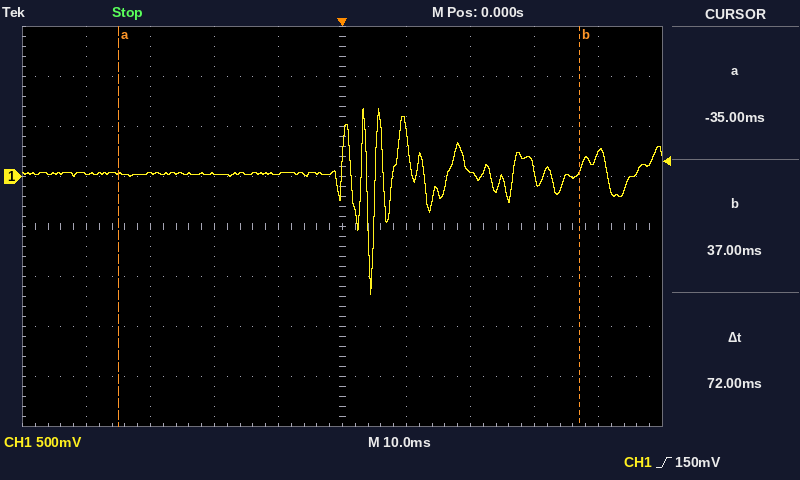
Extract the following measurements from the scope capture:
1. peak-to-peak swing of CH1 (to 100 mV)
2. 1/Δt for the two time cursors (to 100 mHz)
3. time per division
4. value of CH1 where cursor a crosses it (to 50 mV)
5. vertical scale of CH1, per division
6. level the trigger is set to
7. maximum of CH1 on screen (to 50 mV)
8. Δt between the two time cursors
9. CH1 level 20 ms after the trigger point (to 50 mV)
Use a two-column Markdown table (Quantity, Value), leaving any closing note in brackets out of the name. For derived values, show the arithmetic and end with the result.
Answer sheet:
| Quantity | Value |
|---|---|
| peak-to-peak swing of CH1 | 1.90 V |
| 1/Δt for the two time cursors | 1 / 72 ms ≈ 13.9 Hz |
| time per division | 10 ms |
| value of CH1 where cursor a crosses it | 50 mV |
| vertical scale of CH1, per division | 500 mV |
| level the trigger is set to | 150 mV |
| maximum of CH1 on screen | 700 mV |
| Δt between the two time cursors | 72 ms |
| CH1 level 20 ms after the trigger point | 50 mV |
